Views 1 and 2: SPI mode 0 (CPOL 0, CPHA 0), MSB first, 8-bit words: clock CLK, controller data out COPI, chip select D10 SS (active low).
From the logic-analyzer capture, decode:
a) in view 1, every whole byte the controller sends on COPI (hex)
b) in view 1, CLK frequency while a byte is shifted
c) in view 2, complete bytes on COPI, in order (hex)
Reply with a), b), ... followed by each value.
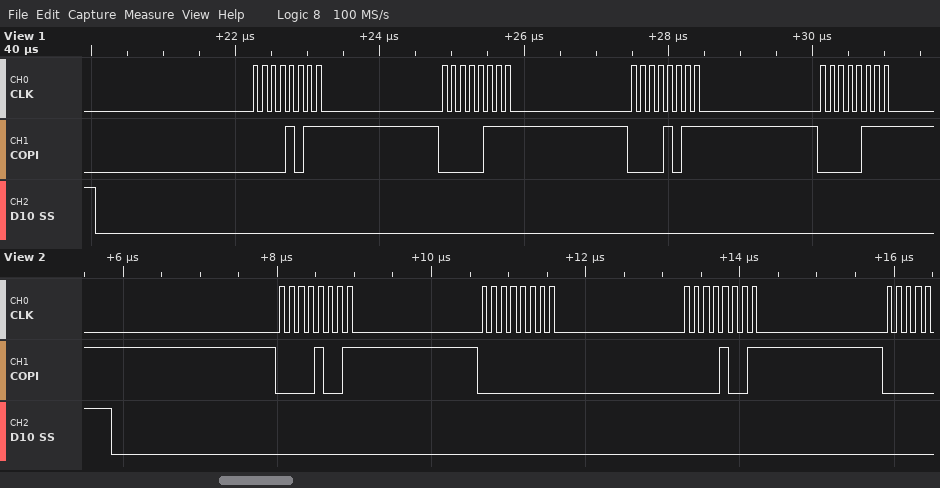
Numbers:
a) 0B 07 0B 07
b) 8 MHz
c) 09 00 09
